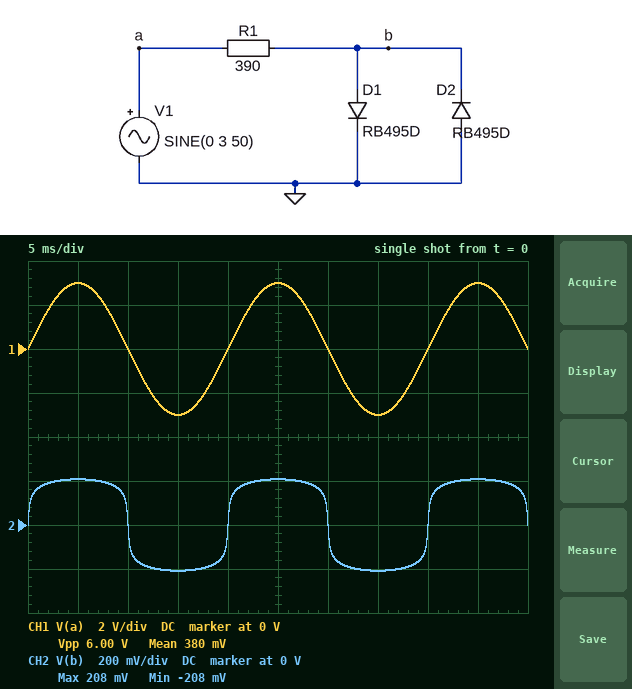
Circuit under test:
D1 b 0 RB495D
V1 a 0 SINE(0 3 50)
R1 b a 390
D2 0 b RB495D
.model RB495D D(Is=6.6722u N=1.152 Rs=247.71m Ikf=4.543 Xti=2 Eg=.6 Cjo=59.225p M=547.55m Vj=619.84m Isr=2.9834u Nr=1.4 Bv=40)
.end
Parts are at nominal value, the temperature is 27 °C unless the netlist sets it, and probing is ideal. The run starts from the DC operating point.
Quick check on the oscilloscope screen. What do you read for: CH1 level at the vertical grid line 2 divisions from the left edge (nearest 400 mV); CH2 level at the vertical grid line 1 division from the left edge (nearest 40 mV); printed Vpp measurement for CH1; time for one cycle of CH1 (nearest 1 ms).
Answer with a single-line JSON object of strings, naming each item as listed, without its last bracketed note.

{"CH1 level at the vertical grid line 2 divisions from the left edge": "0 V", "CH2 level at the vertical grid line 1 division from the left edge": "200 mV", "printed Vpp measurement for CH1": "6.00 V", "time for one cycle of CH1": "20 ms"}
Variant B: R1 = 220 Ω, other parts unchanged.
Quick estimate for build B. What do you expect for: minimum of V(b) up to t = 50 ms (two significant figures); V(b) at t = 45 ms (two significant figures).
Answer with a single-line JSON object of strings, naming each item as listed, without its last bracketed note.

{"minimum of V(b) up to t = 50 ms": "-230 mV", "V(b) at t = 45 ms": "230 mV"}
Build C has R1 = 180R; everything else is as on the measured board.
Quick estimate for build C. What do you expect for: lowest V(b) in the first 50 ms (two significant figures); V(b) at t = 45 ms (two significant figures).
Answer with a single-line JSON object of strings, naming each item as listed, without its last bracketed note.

{"lowest V(b) in the first 50 ms": "-230 mV", "V(b) at t = 45 ms": "230 mV"}
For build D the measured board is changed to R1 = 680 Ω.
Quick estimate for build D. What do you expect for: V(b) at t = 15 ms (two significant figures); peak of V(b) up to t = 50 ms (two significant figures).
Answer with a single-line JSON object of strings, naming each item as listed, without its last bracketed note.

{"V(b) at t = 15 ms": "-190 mV", "peak of V(b) up to t = 50 ms": "190 mV"}
